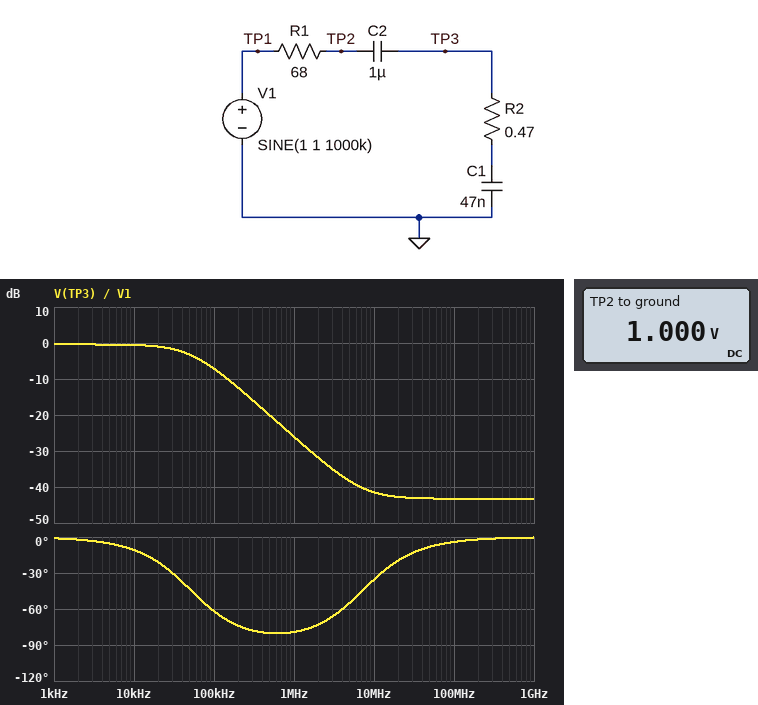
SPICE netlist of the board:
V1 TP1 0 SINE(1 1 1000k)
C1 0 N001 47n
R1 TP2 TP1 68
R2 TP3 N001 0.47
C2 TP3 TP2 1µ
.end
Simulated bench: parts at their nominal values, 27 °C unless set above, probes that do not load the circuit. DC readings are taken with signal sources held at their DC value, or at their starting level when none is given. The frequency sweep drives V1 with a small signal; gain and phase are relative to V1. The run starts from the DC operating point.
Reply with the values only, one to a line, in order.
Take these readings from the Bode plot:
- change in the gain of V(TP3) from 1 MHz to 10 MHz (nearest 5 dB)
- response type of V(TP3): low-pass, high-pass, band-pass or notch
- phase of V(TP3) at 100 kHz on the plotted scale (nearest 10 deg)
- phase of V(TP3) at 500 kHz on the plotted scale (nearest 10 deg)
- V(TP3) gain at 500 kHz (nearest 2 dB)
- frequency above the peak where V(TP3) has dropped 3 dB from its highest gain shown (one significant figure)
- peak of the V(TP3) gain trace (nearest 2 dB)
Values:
-15 dB
low-pass
-60 deg
-80 deg
-20 dB
50 kHz
0 dB
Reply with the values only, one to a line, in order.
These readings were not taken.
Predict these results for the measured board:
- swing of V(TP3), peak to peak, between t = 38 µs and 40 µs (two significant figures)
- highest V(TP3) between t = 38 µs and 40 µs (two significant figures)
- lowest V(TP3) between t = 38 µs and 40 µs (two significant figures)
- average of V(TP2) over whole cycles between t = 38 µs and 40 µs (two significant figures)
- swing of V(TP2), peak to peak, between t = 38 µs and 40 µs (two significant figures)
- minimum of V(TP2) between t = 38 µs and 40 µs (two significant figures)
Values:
100 mV
50 mV
-50 mV
1.0 V
100 mV
950 mV
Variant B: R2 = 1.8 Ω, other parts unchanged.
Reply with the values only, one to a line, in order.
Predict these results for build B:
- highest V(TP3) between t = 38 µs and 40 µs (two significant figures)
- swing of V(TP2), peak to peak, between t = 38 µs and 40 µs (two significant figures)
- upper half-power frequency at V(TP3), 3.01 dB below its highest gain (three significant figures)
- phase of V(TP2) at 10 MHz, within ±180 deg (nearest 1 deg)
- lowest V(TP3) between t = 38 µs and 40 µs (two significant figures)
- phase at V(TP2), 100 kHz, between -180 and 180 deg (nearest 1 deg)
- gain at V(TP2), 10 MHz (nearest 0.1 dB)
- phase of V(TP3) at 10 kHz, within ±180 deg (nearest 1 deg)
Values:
55 mV
110 mV
50.8 kHz
-11 deg
-55 mV
-60 deg
-31.6 dB
-11 deg
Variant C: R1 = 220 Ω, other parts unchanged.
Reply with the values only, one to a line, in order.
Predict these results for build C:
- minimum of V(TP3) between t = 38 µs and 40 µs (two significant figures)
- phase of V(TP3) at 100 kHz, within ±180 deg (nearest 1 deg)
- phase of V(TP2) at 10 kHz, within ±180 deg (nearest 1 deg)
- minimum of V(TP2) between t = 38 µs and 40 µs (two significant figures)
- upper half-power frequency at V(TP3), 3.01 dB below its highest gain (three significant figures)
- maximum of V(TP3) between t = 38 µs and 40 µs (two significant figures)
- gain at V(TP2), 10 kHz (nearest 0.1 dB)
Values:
-15 mV
-80 deg
-32 deg
980 mV
16.1 kHz
16 mV
-1.4 dB
